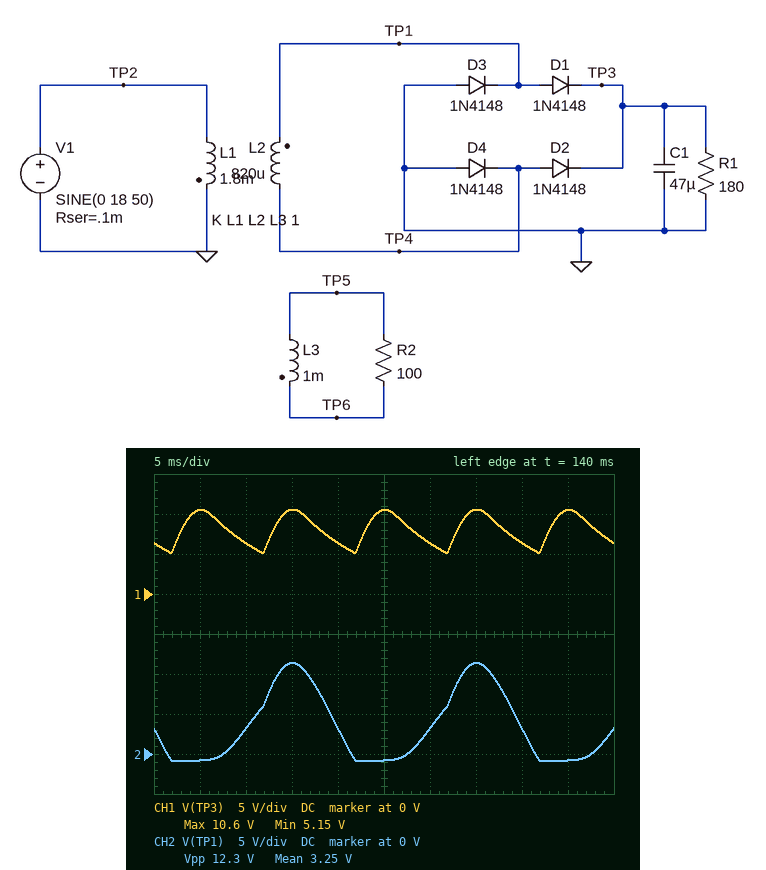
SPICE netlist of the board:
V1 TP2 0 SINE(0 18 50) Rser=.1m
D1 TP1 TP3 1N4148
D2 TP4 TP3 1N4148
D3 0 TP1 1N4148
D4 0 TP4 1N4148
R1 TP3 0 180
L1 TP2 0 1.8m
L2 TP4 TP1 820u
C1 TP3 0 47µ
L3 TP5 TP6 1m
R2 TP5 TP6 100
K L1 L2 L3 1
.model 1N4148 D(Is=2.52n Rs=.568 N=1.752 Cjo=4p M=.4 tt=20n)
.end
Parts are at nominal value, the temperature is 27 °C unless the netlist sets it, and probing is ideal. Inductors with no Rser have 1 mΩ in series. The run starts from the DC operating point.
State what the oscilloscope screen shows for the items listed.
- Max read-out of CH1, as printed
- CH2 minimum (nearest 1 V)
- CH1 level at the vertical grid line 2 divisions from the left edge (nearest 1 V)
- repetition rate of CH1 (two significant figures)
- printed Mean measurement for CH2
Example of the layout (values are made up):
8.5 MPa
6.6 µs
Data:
10.6 V
-1 V
6 V
100 Hz
3.25 V
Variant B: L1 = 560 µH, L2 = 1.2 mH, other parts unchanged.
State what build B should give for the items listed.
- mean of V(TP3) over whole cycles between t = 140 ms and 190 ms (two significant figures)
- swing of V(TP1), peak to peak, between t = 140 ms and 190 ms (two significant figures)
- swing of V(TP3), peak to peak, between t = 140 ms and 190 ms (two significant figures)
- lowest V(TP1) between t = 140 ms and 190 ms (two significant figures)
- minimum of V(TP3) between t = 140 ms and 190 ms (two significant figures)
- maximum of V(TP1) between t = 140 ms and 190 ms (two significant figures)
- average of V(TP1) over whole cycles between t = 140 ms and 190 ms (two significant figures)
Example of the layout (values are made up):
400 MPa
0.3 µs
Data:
19 V
27 V
13 V
-1.1 V
12 V
26 V
9.5 V
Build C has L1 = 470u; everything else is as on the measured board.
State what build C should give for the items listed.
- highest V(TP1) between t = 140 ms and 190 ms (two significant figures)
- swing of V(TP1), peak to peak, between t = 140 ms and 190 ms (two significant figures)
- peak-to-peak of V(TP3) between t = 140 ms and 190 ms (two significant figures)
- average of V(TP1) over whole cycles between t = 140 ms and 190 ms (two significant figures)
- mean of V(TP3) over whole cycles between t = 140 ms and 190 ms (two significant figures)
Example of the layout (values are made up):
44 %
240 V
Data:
23 V
24 V
11 V
8.5 V
17 V
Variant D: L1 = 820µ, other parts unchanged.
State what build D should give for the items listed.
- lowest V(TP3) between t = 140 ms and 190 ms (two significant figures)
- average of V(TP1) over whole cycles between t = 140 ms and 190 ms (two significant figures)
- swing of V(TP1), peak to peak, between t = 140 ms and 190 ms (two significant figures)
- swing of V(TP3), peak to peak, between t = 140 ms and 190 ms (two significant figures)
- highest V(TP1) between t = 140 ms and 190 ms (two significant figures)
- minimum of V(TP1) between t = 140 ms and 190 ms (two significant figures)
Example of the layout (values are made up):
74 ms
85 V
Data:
8.0 V
6.3 V
18 V
8.4 V
17 V
-980 mV
